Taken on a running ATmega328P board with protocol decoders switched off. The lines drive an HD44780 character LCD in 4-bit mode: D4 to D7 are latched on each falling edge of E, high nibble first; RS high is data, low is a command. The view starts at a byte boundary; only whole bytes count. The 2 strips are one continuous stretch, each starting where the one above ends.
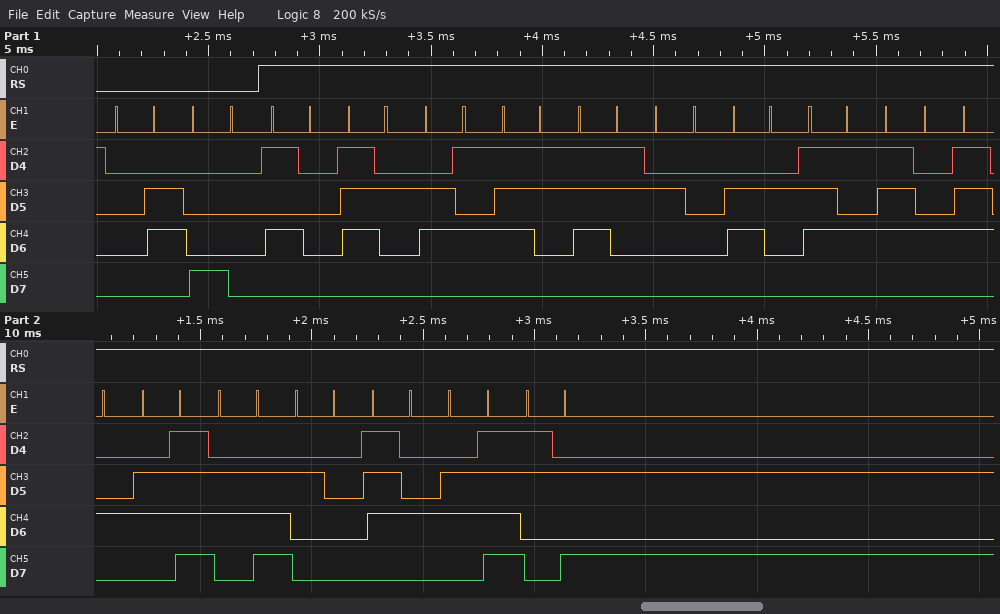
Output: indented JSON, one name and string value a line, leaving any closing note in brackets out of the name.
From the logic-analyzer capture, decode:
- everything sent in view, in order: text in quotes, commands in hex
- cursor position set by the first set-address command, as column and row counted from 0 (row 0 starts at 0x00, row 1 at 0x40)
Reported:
{
  "everything sent in view, in order: text in quotes, commands in hex": "0x06 0x80 \"Press button to:\"",
  "cursor position set by the first set-address command, as column and row counted from 0": "column 0, row 0"
}
